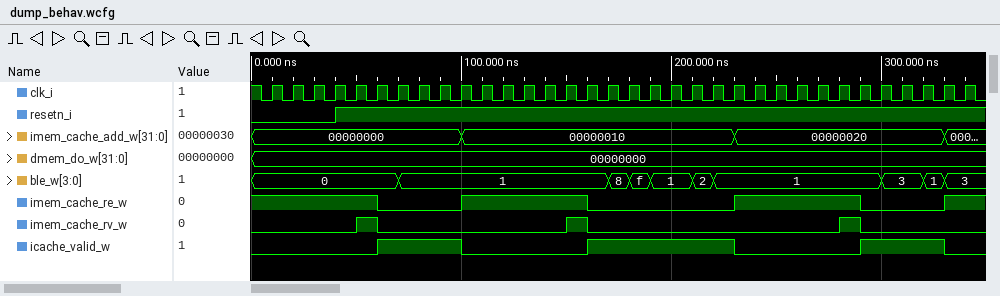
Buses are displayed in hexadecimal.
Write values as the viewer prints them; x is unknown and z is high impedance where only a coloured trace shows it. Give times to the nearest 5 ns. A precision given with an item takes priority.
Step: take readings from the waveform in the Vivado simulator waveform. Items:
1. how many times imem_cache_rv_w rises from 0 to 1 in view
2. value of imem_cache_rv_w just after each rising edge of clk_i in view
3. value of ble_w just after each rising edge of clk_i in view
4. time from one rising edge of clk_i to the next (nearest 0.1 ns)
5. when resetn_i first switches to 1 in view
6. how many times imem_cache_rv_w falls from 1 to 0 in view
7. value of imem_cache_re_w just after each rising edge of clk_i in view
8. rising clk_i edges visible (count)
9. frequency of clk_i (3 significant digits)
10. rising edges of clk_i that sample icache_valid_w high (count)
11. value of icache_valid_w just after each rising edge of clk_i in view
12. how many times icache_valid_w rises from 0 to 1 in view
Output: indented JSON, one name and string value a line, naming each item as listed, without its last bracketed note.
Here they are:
{
  "how many times imem_cache_rv_w rises from 0 to 1 in view": "3",
  "value of imem_cache_rv_w just after each rising edge of clk_i in view": "0 0 0 0 1 0 0 0 0 0 0 0 0 0 1 0 0 0 0 0 0 0 0 0 0 0 0 1 0 0 0 0 0 0",
  "value of ble_w just after each rising edge of clk_i in view": "0, 0, 0, 0, 0, 0, 1, 1, 1, 1, 1, 1, 1, 1, 1, 1, 8, f, 1, 1, 2, 1, 1, 1, 1, 1, 1, 1, 1, 3, 3, 1, 3, 3",
  "time from one rising edge of clk_i to the next": "10 ns",
  "when resetn_i first switches to 1 in view": "40 ns",
  "how many times imem_cache_rv_w falls from 1 to 0 in view": "3",
  "value of imem_cache_re_w just after each rising edge of clk_i in view": "1 1 1 1 1 0 0 0 0 1 1 1 1 1 1 0 0 0 0 0 0 0 1 1 1 1 1 1 0 0 0 0 1 1",
  "rising clk_i edges visible": "34",
  "frequency of clk_i": "100 MHz",
  "rising edges of clk_i that sample icache_valid_w high": "15",
  "value of icache_valid_w just after each rising edge of clk_i in view": "0 0 0 0 0 1 1 1 1 0 0 0 0 0 0 1 1 1 1 1 1 1 0 0 0 0 0 0 1 1 1 1 0 0",
  "how many times icache_valid_w rises from 0 to 1 in view": "3"
}
